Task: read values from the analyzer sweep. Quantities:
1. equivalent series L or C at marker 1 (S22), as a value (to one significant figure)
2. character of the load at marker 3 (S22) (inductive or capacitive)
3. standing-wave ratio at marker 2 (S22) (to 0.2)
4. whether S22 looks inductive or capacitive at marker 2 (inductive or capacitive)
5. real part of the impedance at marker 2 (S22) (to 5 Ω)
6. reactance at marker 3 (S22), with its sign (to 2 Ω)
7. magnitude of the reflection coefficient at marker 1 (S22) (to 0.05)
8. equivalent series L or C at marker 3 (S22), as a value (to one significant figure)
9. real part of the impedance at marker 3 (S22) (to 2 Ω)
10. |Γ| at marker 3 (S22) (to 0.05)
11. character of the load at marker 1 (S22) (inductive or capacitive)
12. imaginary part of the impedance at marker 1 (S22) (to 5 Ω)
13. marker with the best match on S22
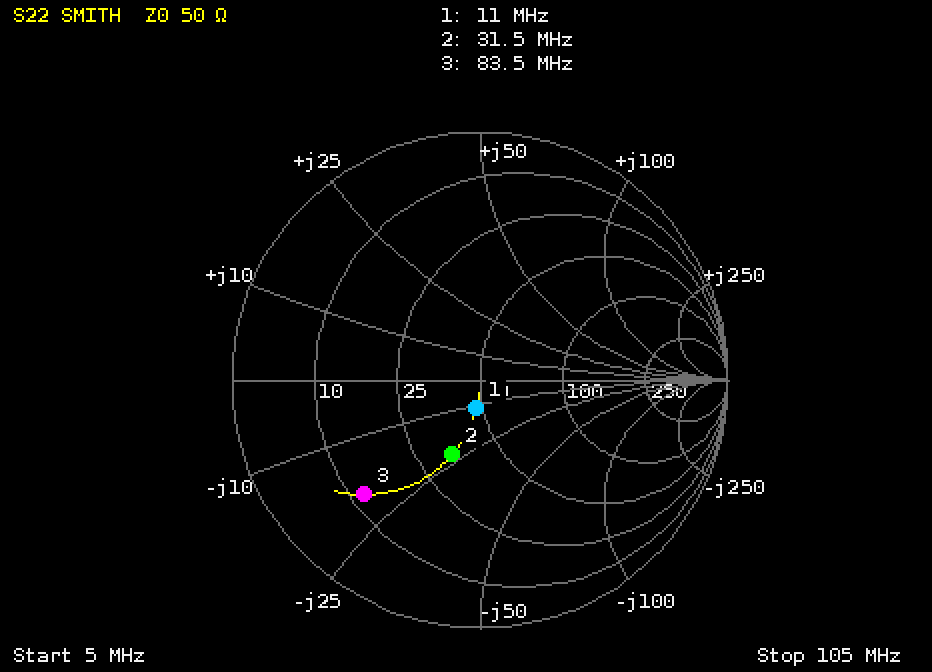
1 nF
capacitive
2.0
capacitive
35 Ω
-20 Ω
0.10
100 pF
12 Ω
0.65
capacitive
-10 Ω
marker 1
